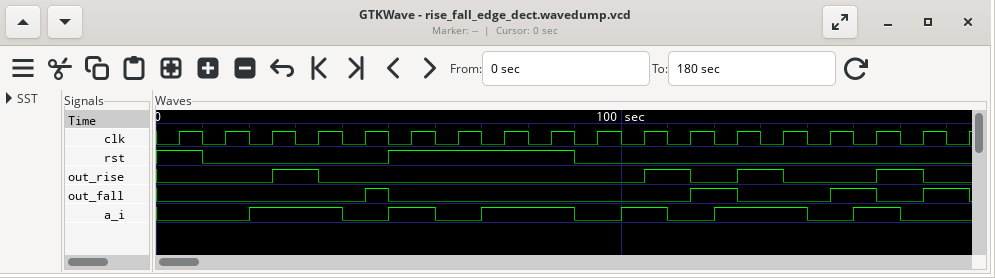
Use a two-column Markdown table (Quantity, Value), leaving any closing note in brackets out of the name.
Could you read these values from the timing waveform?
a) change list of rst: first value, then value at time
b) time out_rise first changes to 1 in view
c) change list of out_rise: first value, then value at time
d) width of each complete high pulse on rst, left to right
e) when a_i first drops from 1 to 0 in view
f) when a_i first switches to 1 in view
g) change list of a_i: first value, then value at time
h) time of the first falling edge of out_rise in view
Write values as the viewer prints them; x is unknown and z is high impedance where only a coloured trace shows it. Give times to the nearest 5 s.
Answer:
| Quantity | Value |
|---|---|
| change list of rst: first value, then value at time | 1, 0 at 10 s, 1 at 50 s, 0 at 90 s |
| time out_rise first changes to 1 in view | 25 s |
| change list of out_rise: first value, then value at time | 0, 1 at 25 s, 0 at 35 s, 1 at 105 s, 0 at 115 s, 1 at 125 s, 0 at 135 s, 1 at 155 s, 0 at 165 s |
| width of each complete high pulse on rst, left to right | 40 s |
| when a_i first drops from 1 to 0 in view | 40 s |
| when a_i first switches to 1 in view | 20 s |
| change list of a_i: first value, then value at time | 0, 1 at 20 s, 0 at 40 s, 1 at 50 s, 0 at 60 s, 1 at 70 s, 0 at 90 s, 1 at 100 s, 0 at 110 s, 1 at 120 s, 0 at 140 s, 1 at 150 s, 0 at 160 s |
| time of the first falling edge of out_rise in view | 35 s |
